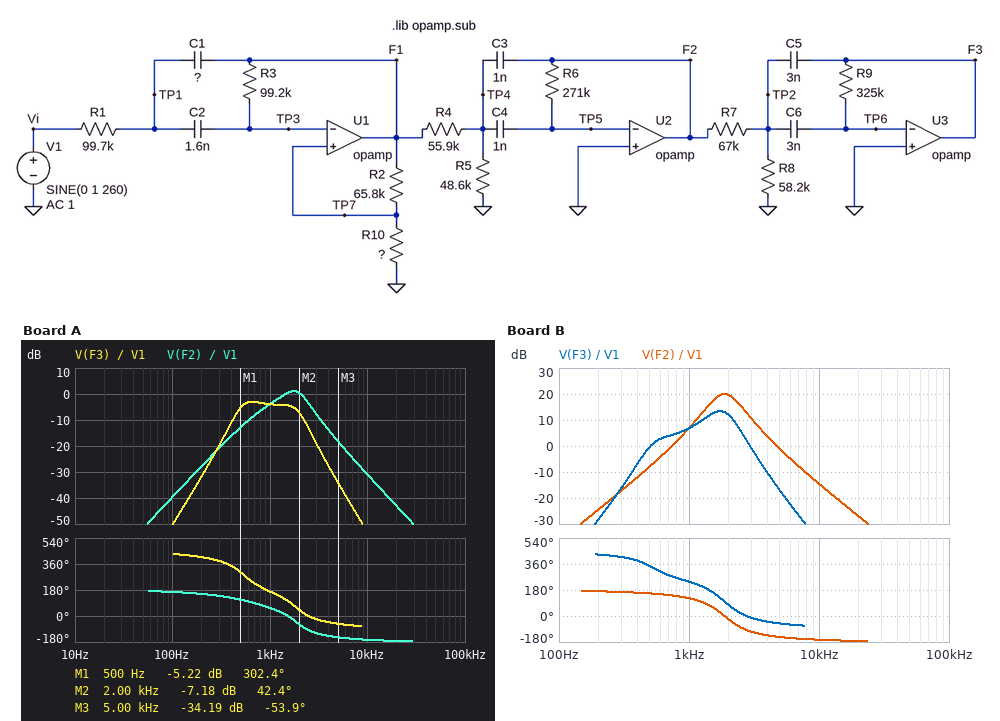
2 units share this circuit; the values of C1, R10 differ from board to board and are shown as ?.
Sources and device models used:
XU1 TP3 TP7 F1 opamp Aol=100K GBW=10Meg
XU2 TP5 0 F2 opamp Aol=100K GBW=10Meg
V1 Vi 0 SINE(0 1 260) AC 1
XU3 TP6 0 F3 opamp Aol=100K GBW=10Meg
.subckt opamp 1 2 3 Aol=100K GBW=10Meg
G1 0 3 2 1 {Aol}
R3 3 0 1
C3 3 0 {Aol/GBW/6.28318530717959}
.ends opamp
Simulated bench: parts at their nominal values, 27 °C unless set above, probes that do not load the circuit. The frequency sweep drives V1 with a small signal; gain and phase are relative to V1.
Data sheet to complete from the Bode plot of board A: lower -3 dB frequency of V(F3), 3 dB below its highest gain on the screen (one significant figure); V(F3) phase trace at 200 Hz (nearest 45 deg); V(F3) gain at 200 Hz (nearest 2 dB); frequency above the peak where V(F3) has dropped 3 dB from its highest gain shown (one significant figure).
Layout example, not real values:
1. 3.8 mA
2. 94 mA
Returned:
1. 500 Hz
2. 405 deg
3. -32 dB
4. 2 kHz
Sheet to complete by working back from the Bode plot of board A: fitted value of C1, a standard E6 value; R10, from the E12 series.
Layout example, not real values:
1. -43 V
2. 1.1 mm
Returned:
1. 2.2 nF
2. 22 kΩ
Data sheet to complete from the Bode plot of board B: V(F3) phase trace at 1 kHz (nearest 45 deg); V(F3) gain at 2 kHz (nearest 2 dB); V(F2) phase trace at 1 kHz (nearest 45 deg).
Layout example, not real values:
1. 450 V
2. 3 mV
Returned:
1. 225 deg
2. 12 dB
3. 135 deg
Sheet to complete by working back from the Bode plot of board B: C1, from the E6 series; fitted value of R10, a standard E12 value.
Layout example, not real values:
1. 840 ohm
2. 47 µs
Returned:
1. 470 pF
2. 56 kΩ
